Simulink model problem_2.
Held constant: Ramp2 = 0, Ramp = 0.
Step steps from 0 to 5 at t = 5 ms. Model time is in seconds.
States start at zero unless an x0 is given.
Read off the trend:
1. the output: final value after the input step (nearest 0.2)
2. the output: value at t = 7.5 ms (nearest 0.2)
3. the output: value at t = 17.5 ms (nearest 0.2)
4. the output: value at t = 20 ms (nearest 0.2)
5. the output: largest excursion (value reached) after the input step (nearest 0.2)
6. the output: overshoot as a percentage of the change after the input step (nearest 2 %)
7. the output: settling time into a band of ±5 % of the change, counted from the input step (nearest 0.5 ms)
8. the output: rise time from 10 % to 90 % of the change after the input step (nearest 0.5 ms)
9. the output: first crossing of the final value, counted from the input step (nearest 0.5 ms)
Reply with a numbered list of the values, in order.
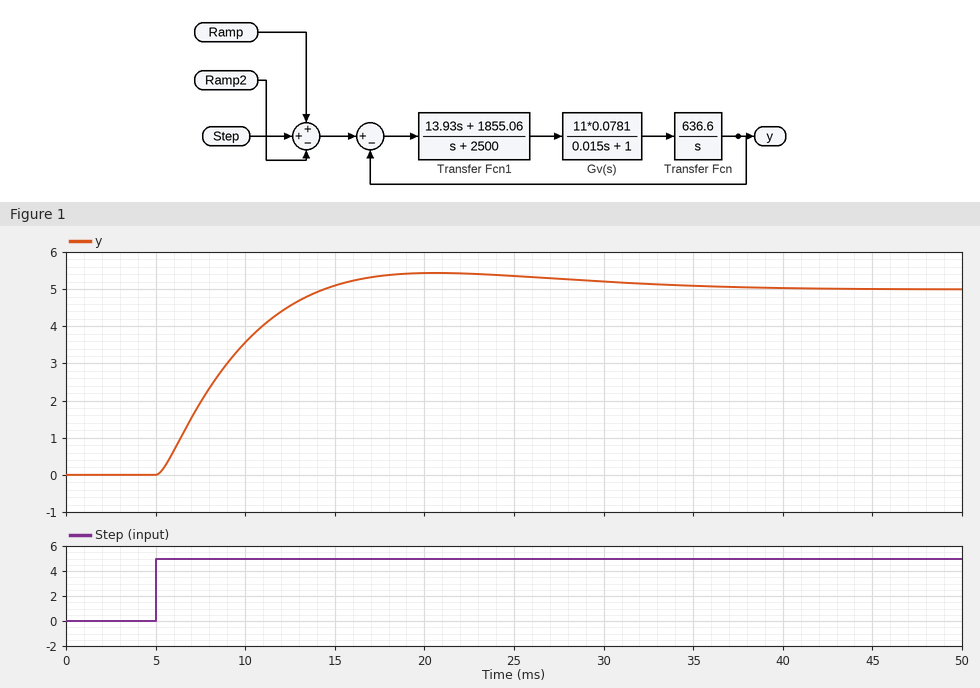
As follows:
1. 5.0
2. 2.0
3. 5.4
4. 5.4
5. 5.4
6. 8 %
7. 23.5 ms
8. 6.5 ms
9. 9.5 ms
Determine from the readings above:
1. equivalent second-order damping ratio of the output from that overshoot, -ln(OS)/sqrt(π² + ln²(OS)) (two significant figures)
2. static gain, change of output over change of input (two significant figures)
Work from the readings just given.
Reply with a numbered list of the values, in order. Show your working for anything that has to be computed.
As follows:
1. ln(0.08) = -2.526; 2.526 / sqrt(9.870 + 6.379) = 0.63
2. (5 - 0) / (5 - 0) = 1.0
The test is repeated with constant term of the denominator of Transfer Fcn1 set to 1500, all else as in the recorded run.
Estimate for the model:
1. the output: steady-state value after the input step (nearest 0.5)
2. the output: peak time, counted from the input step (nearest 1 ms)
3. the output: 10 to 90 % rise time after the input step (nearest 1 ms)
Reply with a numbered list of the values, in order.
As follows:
1. 5.0
2. 10 ms
3. 4 ms
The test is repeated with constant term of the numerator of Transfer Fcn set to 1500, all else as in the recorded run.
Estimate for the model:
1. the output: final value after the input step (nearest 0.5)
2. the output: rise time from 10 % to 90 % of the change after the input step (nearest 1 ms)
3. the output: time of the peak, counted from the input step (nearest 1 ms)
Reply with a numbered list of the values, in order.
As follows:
1. 5.0
2. 3 ms
3. 8 ms
